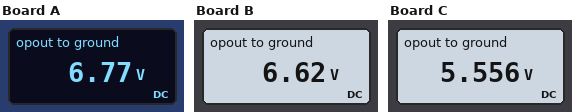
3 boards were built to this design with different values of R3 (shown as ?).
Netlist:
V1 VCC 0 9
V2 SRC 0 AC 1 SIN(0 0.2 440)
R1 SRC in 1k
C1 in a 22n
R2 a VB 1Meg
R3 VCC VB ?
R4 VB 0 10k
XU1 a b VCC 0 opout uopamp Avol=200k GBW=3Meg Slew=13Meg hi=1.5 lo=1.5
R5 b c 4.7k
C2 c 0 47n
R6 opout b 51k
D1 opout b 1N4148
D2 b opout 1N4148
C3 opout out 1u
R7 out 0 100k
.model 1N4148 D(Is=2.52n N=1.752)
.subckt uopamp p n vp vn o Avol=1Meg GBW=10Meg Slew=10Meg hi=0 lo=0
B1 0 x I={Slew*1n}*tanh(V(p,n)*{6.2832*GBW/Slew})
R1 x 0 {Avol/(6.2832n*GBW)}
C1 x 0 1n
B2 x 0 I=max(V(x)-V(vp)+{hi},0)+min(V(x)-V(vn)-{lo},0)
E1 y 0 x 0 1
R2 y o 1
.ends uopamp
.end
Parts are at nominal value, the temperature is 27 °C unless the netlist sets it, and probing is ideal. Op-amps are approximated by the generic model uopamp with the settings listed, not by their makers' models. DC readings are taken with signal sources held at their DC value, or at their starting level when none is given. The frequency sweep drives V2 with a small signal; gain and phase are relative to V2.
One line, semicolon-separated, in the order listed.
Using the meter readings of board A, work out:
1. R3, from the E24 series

3.3 kΩ
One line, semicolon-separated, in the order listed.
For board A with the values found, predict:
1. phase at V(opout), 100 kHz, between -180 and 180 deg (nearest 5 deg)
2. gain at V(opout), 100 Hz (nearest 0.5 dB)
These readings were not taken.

-20 deg; 5.5 dB
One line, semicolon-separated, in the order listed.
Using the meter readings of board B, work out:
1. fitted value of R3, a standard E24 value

3.6 kΩ
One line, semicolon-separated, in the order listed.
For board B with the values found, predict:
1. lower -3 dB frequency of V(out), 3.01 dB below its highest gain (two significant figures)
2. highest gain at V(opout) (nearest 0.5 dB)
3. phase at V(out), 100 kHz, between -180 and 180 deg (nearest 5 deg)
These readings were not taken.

710 Hz; 21.5 dB; -20 deg
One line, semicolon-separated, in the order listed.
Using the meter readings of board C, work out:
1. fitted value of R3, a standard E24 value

6.2 kΩ
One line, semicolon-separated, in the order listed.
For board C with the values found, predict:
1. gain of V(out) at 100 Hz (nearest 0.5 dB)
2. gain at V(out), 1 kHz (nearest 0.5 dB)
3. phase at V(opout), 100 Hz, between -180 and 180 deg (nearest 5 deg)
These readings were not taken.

5.5 dB; 19.5 dB; 55 deg
